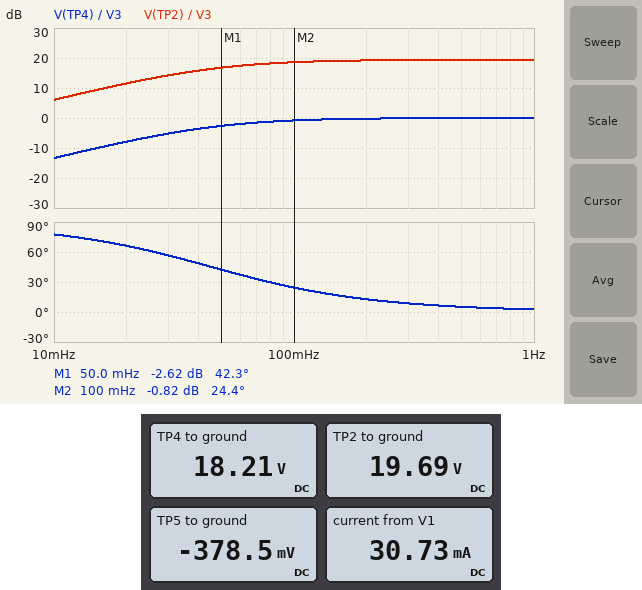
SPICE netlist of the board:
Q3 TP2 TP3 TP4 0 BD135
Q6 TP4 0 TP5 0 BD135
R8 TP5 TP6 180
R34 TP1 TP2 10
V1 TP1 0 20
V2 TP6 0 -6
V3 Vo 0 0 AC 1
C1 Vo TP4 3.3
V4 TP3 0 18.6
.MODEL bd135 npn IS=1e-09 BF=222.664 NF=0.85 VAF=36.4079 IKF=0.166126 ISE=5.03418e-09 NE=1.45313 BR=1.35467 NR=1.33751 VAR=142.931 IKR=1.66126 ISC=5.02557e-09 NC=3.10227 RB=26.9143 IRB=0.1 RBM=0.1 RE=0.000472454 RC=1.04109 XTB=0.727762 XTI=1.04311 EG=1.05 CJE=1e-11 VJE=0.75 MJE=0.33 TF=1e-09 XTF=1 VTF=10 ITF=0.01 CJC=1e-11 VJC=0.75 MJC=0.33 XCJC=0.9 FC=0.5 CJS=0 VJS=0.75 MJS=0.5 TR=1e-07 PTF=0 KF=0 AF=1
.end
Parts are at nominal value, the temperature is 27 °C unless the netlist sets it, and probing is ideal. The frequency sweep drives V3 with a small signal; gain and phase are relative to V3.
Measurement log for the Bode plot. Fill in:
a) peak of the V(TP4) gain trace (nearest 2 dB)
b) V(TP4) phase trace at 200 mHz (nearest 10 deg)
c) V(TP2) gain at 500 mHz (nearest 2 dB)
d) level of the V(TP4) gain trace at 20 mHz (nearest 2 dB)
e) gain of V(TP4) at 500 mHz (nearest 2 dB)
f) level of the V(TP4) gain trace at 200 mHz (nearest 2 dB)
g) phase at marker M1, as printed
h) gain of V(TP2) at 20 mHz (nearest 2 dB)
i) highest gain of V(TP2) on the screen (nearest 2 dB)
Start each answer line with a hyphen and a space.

- 0 dB
- 10 deg
- 20 dB
- -8 dB
- 0 dB
- 0 dB
- 42.3 deg
- 12 dB
- 20 dB
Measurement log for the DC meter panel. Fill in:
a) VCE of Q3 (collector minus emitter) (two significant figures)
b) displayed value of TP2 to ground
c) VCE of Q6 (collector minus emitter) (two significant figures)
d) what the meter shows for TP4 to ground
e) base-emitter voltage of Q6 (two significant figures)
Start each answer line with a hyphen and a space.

- 1.5 V
- 19.69 V
- 19 V
- 18.21 V
- 380 mV
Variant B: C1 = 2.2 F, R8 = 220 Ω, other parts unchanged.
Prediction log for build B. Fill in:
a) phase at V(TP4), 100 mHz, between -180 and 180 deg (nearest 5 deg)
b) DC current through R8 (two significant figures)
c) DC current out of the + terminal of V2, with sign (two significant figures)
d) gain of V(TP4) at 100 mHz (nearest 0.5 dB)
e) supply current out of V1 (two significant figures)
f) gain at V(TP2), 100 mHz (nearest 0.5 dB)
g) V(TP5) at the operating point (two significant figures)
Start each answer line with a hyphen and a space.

- 30 deg
- 26 mA
- -26 mA
- -1.5 dB
- 25 mA
- 17.0 dB
- -370 mV
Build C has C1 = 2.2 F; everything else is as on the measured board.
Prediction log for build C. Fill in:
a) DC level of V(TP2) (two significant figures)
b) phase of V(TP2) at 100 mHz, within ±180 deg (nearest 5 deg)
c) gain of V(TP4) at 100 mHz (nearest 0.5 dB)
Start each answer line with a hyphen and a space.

- 20 V
- 35 deg
- -1.5 dB
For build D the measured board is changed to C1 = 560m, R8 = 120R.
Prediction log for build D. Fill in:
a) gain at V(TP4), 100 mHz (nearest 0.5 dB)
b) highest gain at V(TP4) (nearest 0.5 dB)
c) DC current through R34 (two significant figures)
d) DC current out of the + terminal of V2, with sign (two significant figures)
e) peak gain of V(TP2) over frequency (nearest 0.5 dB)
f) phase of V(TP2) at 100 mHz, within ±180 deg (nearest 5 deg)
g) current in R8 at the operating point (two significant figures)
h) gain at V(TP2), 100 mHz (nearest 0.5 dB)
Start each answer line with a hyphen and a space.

- -11.0 dB
- 0 dB
- 46 mA
- -47 mA
- 21.5 dB
- 75 deg
- 47 mA
- 10.5 dB
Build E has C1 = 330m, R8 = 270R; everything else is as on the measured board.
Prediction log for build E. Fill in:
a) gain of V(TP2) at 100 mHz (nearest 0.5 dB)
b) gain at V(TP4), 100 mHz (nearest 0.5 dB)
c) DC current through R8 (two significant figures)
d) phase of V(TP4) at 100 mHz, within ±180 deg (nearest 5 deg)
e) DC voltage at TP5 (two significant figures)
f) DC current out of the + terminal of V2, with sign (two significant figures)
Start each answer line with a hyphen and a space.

- 6.0 dB
- -11.0 dB
- 21 mA
- 75 deg
- -370 mV
- -21 mA
